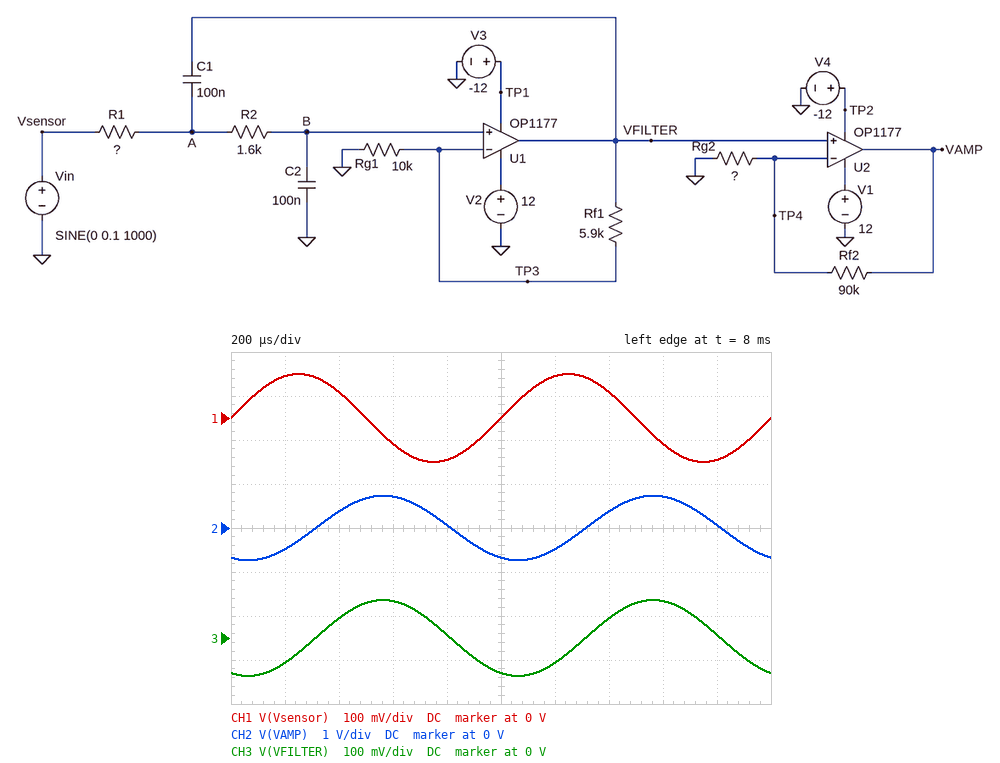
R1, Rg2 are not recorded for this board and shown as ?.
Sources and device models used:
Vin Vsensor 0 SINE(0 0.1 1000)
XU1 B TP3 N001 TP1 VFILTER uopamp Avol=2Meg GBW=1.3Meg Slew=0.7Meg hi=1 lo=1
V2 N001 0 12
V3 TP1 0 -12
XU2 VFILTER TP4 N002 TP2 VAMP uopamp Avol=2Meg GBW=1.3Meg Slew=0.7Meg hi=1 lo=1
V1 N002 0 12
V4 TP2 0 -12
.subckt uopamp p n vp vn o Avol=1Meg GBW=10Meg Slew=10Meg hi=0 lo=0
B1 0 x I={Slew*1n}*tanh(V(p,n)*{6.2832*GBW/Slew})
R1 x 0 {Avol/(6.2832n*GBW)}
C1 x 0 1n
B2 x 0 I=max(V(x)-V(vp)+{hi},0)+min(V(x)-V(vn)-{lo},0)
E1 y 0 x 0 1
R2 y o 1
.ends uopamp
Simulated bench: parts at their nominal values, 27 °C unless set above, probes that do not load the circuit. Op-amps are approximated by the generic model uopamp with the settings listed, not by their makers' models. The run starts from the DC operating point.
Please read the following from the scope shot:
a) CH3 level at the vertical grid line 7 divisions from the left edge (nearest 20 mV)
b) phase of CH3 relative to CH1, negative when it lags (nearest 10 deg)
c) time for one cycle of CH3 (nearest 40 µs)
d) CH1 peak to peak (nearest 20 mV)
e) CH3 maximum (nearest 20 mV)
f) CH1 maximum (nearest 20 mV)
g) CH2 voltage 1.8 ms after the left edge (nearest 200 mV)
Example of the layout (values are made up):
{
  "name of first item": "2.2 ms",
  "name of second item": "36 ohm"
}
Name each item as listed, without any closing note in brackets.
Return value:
{
  "CH3 level at the vertical grid line 7 divisions from the left edge": "40 mV",
  "phase of CH3 relative to CH1, negative when it lags": "-110 deg",
  "time for one cycle of CH3": "1.00 ms",
  "CH1 peak to peak": "200 mV",
  "CH3 maximum": "80 mV",
  "CH1 maximum": "100 mV",
  "CH2 voltage 1.8 ms after the left edge": "0 V"
}
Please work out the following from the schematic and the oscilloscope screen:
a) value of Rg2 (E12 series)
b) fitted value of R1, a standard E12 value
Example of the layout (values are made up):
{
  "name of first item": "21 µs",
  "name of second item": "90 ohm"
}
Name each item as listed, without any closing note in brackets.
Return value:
{
  "value of Rg2": "12 kΩ",
  "fitted value of R1, a standard E12 value": "2.7 kΩ"
}
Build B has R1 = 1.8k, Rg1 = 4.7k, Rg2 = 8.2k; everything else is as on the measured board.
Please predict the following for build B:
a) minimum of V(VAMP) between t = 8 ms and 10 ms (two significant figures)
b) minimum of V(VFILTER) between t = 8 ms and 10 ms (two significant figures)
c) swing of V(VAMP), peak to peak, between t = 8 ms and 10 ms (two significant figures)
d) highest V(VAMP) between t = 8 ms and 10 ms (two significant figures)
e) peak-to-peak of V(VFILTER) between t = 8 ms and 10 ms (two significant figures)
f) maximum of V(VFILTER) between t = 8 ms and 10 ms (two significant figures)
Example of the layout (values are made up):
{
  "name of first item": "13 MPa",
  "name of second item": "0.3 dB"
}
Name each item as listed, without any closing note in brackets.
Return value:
{
  "minimum of V(VAMP) between t = 8 ms and 10 ms": "-3.7 V",
  "minimum of V(VFILTER) between t = 8 ms and 10 ms": "-310 mV",
  "swing of V(VAMP), peak to peak, between t = 8 ms and 10 ms": "7.4 V",
  "highest V(VAMP) between t = 8 ms and 10 ms": "3.7 V",
  "peak-to-peak of V(VFILTER) between t = 8 ms and 10 ms": "620 mV",
  "maximum of V(VFILTER) between t = 8 ms and 10 ms": "310 mV"
}
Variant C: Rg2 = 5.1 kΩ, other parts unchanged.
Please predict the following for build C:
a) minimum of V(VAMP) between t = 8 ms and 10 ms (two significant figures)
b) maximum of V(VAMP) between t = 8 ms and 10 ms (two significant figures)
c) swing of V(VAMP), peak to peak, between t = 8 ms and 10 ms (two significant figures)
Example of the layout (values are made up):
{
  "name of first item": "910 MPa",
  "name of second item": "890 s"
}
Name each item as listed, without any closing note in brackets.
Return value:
{
  "minimum of V(VAMP) between t = 8 ms and 10 ms": "-1.6 V",
  "maximum of V(VAMP) between t = 8 ms and 10 ms": "1.6 V",
  "swing of V(VAMP), peak to peak, between t = 8 ms and 10 ms": "3.2 V"
}
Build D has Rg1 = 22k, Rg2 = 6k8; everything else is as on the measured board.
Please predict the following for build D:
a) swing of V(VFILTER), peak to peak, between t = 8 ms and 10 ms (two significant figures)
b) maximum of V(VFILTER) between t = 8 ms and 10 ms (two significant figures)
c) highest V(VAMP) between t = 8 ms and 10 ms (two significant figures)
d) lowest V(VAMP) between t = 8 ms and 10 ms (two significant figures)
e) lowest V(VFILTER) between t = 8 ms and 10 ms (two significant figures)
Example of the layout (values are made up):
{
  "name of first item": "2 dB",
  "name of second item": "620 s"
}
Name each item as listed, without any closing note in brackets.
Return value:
{
  "swing of V(VFILTER), peak to peak, between t = 8 ms and 10 ms": "110 mV",
  "maximum of V(VFILTER) between t = 8 ms and 10 ms": "54 mV",
  "highest V(VAMP) between t = 8 ms and 10 ms": "770 mV",
  "lowest V(VAMP) between t = 8 ms and 10 ms": "-770 mV",
  "lowest V(VFILTER) between t = 8 ms and 10 ms": "-54 mV"
}
